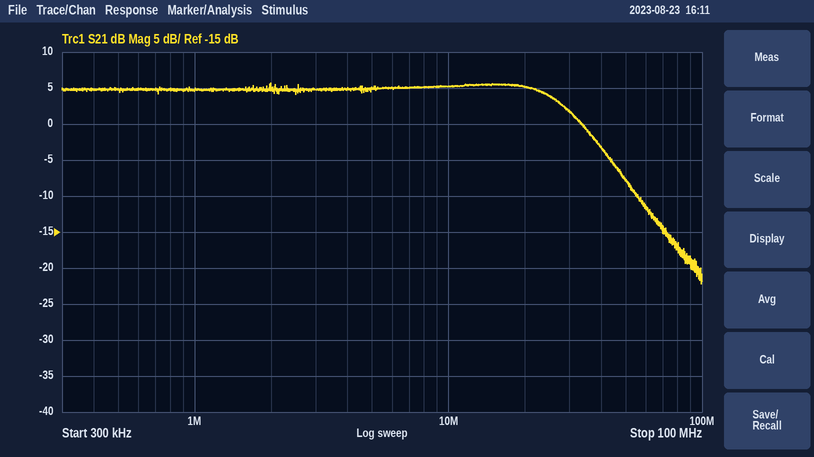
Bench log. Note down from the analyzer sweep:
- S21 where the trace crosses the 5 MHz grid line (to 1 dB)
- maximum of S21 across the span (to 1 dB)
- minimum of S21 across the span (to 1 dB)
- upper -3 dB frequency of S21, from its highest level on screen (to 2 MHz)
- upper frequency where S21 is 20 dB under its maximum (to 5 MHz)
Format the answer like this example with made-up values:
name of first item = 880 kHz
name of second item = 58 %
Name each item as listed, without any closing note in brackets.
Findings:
S21 where the trace crosses the 5 MHz grid line = 5 dB
maximum of S21 across the span = 6 dB
minimum of S21 across the span = -22 dB
upper -3 dB frequency of S21, from its highest level on screen = 28 MHz
upper frequency where S21 is 20 dB under its maximum = 70 MHz
